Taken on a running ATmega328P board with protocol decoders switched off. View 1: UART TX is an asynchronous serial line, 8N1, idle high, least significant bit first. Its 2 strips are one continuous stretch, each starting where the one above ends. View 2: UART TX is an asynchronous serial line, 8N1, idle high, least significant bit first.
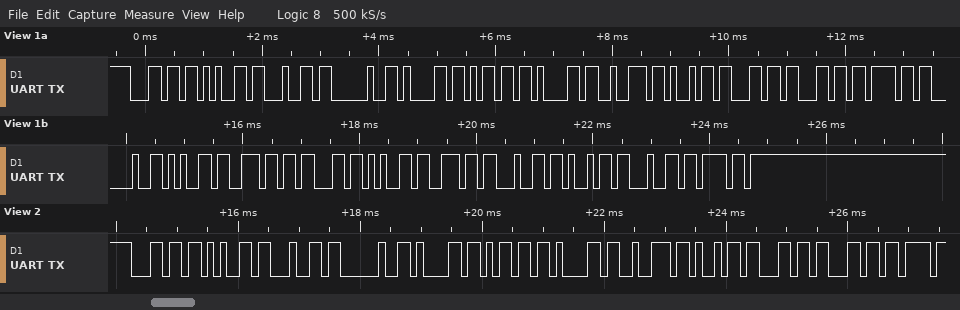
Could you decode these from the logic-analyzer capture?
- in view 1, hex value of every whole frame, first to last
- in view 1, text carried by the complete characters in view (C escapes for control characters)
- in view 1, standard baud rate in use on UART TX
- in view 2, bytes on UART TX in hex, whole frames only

6C 65 64 20 61 6D 61 72 69 6C 6C 6F 20 65 6E 63 65 6E 64 69 64 6F
"led amarillo encendido"
9600 baud
0x6C 0x65 0x64 0x20 0x61 0x6D 0x61 0x72 0x69 0x6C 0x6C
